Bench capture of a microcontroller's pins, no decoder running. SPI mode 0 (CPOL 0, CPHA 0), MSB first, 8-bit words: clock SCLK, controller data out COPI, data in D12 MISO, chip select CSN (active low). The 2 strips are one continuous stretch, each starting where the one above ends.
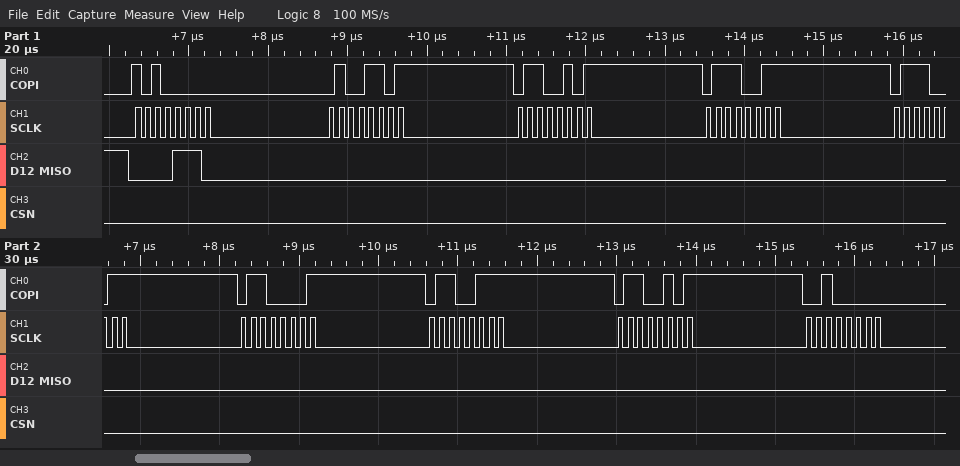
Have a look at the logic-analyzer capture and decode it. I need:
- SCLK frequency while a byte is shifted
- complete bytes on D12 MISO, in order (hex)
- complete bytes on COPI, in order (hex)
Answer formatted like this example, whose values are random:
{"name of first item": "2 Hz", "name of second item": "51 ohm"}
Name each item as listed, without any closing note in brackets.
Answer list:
{"SCLK frequency while a byte is shifted": "8 MHz", "complete bytes on D12 MISO, in order": "0E 00 00 00 00 00 00 00 00", "complete bytes on COPI, in order": "A0 4D 65 73 73 61 67 65 20"}
